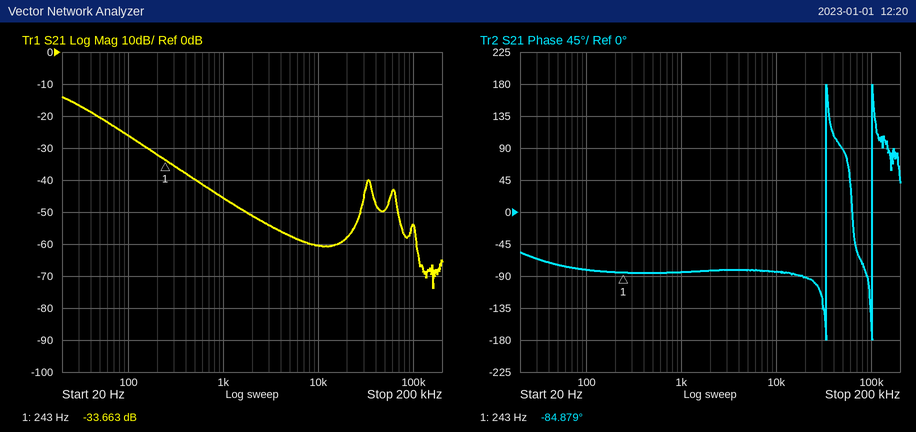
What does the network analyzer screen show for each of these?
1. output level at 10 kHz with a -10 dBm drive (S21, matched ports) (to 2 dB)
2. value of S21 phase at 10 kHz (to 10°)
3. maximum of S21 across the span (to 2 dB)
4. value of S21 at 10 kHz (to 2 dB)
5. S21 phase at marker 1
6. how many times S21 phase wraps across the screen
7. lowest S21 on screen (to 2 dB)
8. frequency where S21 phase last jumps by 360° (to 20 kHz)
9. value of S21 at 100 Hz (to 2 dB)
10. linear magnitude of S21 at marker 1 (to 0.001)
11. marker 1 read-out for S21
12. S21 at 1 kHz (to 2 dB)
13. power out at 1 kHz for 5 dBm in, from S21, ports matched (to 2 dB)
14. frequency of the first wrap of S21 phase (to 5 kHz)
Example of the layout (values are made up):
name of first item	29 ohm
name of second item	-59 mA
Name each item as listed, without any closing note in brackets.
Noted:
output level at 10 kHz with a -10 dBm drive (S21, matched ports)	-70 dBm
value of S21 phase at 10 kHz	-80°
maximum of S21 across the span	-14 dB
value of S21 at 10 kHz	-60 dB
S21 phase at marker 1	-84.879°
how many times S21 phase wraps across the screen	2
lowest S21 on screen	-74 dB
frequency where S21 phase last jumps by 360°	100 kHz
value of S21 at 100 Hz	-26 dB
linear magnitude of S21 at marker 1	0.021
marker 1 read-out for S21	-33.663 dB
S21 at 1 kHz	-46 dB
power out at 1 kHz for 5 dBm in, from S21, ports matched	-40 dBm
frequency of the first wrap of S21 phase	35 kHz
